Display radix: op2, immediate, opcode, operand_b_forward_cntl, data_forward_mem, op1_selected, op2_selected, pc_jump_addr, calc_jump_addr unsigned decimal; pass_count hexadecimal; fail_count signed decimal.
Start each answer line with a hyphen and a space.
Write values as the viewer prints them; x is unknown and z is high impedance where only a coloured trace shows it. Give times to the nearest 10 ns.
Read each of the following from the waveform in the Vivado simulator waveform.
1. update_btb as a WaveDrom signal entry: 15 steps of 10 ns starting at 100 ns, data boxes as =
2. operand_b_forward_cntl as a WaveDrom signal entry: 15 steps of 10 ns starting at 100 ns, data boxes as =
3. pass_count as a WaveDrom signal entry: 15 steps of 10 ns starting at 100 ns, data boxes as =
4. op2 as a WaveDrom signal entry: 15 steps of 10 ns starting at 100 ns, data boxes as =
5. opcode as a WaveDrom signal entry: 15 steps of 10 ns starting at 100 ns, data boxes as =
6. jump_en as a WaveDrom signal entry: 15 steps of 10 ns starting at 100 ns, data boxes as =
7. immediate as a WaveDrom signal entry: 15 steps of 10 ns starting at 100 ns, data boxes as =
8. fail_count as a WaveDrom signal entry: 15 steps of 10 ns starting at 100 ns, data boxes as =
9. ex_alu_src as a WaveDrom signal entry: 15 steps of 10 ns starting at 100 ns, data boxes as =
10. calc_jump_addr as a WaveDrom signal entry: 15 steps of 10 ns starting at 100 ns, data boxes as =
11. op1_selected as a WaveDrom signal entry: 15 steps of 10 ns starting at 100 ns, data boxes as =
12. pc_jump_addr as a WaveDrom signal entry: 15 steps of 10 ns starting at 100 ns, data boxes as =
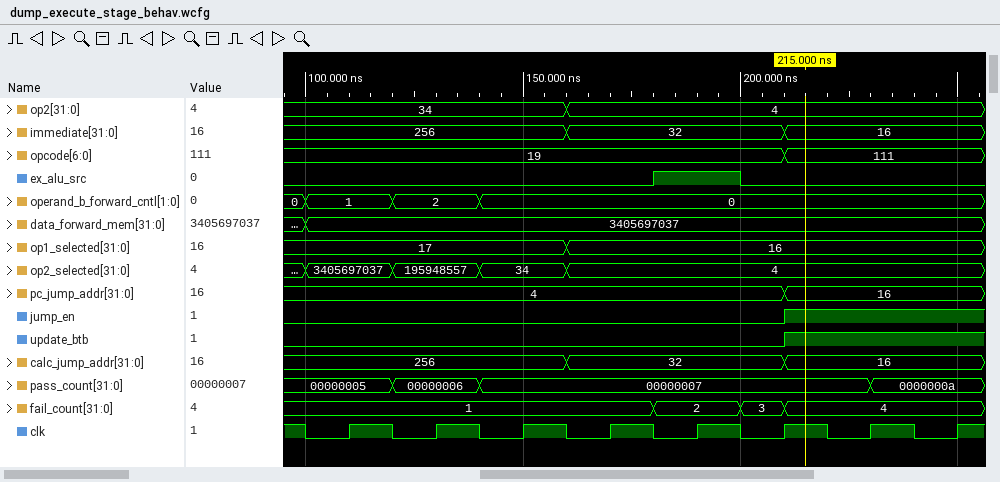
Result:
- {name: 'update_btb', wave: '0..........1...'}
- {name: 'operand_b_forward_cntl', wave: '=.=.=..........', data: '1 2 0'}
- {name: 'pass_count', wave: '=.=.=........=.', data: '00000005 00000006 00000007 0000000a'}
- {name: 'op2', wave: '=.....=........', data: '34 4'}
- {name: 'opcode', wave: '=..........=...', data: '19 111'}
- {name: 'jump_en', wave: '0..........1...'}
- {name: 'immediate', wave: '=.....=....=...', data: '256 32 16'}
- {name: 'fail_count', wave: '=.......=.==...', data: '1 2 3 4'}
- {name: 'ex_alu_src', wave: '0.......1.0....'}
- {name: 'calc_jump_addr', wave: '=.....=....=...', data: '256 32 16'}
- {name: 'op1_selected', wave: '=.....=........', data: '17 16'}
- {name: 'pc_jump_addr', wave: '=..........=...', data: '4 16'}
